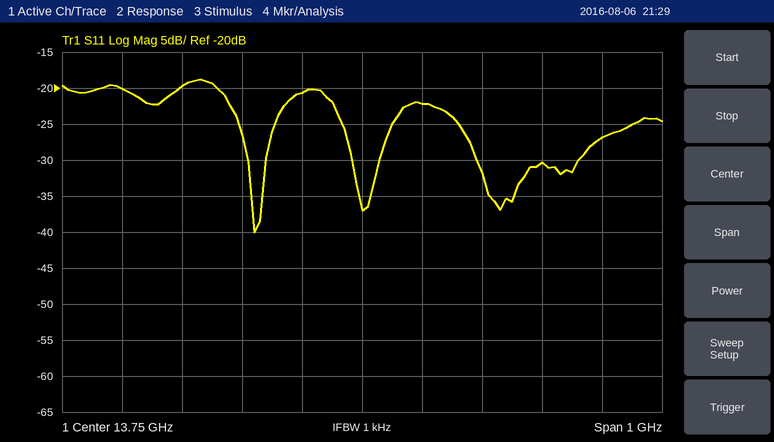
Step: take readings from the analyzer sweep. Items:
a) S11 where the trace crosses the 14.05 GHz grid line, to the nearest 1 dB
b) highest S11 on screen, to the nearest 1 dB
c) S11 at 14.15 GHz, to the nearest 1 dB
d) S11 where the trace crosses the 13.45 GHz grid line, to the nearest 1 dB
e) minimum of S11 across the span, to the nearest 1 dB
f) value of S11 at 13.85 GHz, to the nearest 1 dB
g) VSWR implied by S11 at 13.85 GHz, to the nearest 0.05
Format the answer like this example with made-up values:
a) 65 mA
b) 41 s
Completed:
a) -30 dB
b) -19 dB
c) -27 dB
d) -20 dB
e) -40 dB
f) -22 dB
g) 1.15
